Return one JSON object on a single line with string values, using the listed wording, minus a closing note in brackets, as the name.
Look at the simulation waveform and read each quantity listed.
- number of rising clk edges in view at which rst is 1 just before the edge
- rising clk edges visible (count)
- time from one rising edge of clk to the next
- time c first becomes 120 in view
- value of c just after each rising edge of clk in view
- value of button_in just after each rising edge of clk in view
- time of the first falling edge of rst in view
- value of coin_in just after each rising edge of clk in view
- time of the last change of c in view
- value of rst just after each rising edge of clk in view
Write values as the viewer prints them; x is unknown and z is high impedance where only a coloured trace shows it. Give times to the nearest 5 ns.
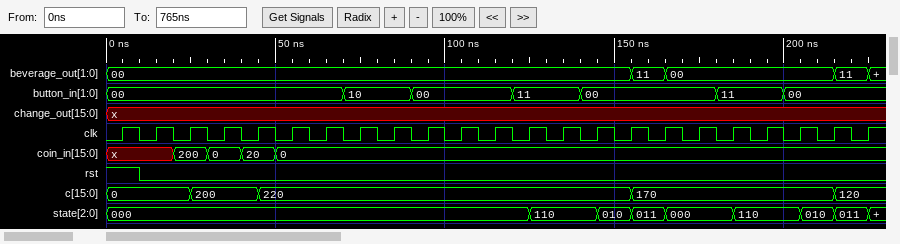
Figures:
{"number of rising clk edges in view at which rst is 1 just before the edge": "1", "rising clk edges visible": "23", "time from one rising edge of clk to the next": "10 ns", "time c first becomes 120 in view": "215 ns", "value of c just after each rising edge of clk in view": "0, 0, 200, 200, 220, 220, 220, 220, 220, 220, 220, 220, 220, 220, 220, 170, 170, 170, 170, 170, 170, 120, 120", "value of button_in just after each rising edge of clk in view": "00, 00, 00, 00, 00, 00, 00, 10, 10, 00, 00, 00, 11, 11, 00, 00, 00, 00, 11, 11, 00, 00, 00", "time of the first falling edge of rst in view": "10 ns", "value of coin_in just after each rising edge of clk in view": "x, x, 200, 0, 20, 0, 0, 0, 0, 0, 0, 0, 0, 0, 0, 0, 0, 0, 0, 0, 0, 0, 0", "time of the last change of c in view": "215 ns", "value of rst just after each rising edge of clk in view": "1 0 0 0 0 0 0 0 0 0 0 0 0 0 0 0 0 0 0 0 0 0 0"}
